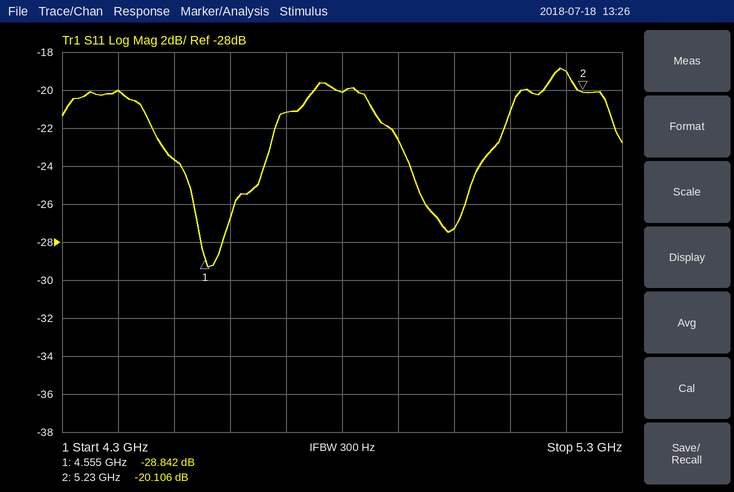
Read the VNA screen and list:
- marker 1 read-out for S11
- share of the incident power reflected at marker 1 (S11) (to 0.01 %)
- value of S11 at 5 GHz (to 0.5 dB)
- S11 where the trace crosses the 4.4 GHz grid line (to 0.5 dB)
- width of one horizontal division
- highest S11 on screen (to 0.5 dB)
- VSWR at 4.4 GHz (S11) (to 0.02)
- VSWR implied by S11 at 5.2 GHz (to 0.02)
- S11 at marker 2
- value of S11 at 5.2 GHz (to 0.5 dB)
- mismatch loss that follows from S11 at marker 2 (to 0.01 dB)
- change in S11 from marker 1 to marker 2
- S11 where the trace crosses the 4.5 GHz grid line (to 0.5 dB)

-28.842 dB
0.13 %
-27.5 dB
-20.0 dB
100 MHz
-19.0 dB
1.22
1.26
-20.106 dB
-19.0 dB
0.04 dB
8.736 dB
-23.5 dB
